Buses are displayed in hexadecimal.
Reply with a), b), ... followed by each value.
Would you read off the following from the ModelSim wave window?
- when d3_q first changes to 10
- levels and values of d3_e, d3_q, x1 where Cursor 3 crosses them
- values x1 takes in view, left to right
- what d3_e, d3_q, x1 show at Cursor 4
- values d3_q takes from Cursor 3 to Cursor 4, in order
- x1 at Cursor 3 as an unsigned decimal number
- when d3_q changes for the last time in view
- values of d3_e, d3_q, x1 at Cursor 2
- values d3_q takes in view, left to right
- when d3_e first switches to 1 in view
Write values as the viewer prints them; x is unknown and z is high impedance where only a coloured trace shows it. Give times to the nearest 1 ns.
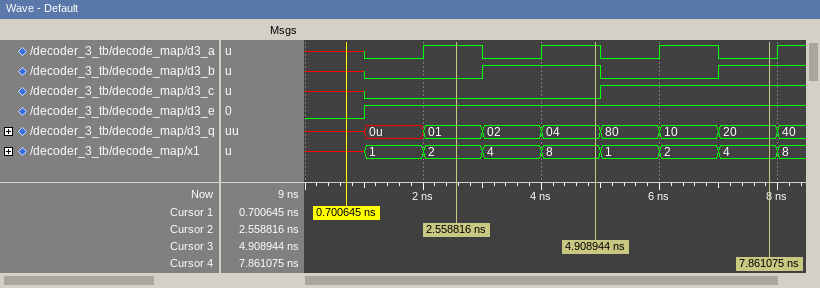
a) 6 ns
b) d3_e=1, d3_q=04, x1=8
c) x, 1, 2, 4, 8, 1, 2, 4, 8
d) d3_e=1, d3_q=20, x1=4
e) 04, 80, 10, 20
f) 8
g) 8 ns
h) d3_e=1, d3_q=01, x1=2
i) x, 0u, 01, 02, 04, 80, 10, 20, 40
j) 1 ns
